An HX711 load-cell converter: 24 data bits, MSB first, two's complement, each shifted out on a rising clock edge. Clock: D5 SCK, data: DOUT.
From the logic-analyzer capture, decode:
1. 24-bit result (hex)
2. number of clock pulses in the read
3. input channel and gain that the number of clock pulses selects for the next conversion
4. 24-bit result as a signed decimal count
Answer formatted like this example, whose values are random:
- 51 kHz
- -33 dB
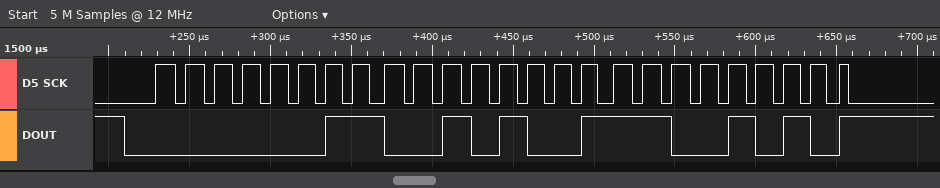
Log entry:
- 0x0329CA
- 25
- channel A, gain 128
- 207306
